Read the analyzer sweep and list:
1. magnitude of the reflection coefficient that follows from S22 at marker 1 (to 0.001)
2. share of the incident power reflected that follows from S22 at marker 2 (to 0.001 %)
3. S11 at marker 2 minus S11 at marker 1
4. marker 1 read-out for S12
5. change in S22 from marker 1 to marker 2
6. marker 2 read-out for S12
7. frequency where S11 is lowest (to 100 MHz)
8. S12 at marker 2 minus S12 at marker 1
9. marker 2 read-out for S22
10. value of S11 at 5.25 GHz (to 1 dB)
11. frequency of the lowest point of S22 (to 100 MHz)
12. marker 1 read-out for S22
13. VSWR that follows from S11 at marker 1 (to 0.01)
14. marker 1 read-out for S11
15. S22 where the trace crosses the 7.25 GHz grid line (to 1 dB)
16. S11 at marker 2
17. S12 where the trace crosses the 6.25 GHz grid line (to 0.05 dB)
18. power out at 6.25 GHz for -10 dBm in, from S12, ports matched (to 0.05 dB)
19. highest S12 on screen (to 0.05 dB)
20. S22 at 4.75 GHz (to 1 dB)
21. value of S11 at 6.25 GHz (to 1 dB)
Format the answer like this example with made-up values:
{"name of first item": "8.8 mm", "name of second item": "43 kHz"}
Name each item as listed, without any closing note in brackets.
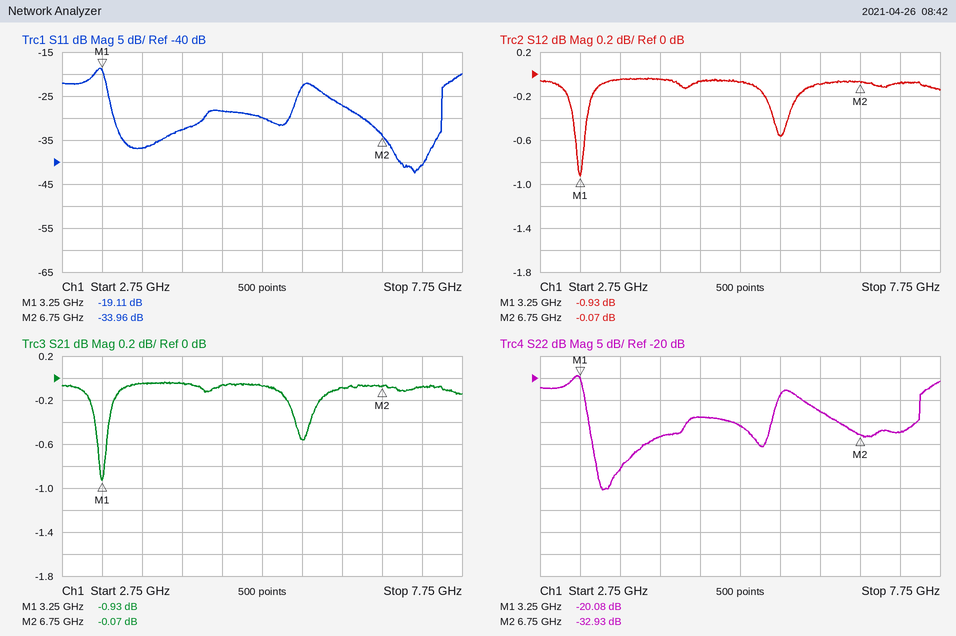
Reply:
{"magnitude of the reflection coefficient that follows from S22 at marker 1": "0.099", "share of the incident power reflected that follows from S22 at marker 2": "0.051 %", "S11 at marker 2 minus S11 at marker 1": "-14.85 dB", "marker 1 read-out for S12": "-0.93 dB", "change in S22 from marker 1 to marker 2": "-12.85 dB", "marker 2 read-out for S12": "-0.07 dB", "frequency where S11 is lowest": "7.2 GHz", "S12 at marker 2 minus S12 at marker 1": "0.86 dB", "marker 2 read-out for S22": "-32.93 dB", "value of S11 at 5.25 GHz": "-30 dB", "frequency of the lowest point of S22": "3.5 GHz", "marker 1 read-out for S22": "-20.08 dB", "VSWR that follows from S11 at marker 1": "1.25", "marker 1 read-out for S11": "-19.11 dB", "S22 where the trace crosses the 7.25 GHz grid line": "-32 dB", "S11 at marker 2": "-33.96 dB", "S12 where the trace crosses the 6.25 GHz grid line": "-0.10 dB", "power out at 6.25 GHz for -10 dBm in, from S12, ports matched": "-10.10 dBm", "highest S12 on screen": "-0.05 dB", "S22 at 4.75 GHz": "-29 dB", "value of S11 at 6.25 GHz": "-27 dB"}
